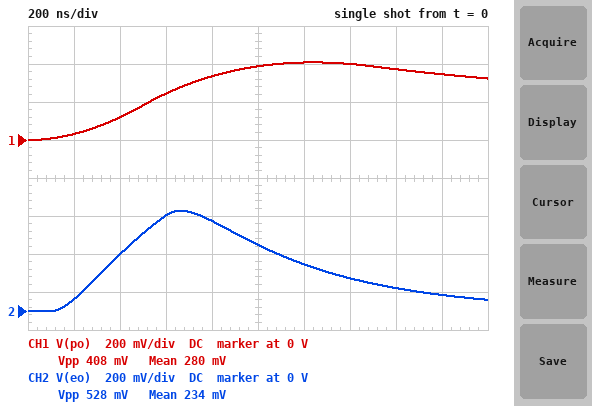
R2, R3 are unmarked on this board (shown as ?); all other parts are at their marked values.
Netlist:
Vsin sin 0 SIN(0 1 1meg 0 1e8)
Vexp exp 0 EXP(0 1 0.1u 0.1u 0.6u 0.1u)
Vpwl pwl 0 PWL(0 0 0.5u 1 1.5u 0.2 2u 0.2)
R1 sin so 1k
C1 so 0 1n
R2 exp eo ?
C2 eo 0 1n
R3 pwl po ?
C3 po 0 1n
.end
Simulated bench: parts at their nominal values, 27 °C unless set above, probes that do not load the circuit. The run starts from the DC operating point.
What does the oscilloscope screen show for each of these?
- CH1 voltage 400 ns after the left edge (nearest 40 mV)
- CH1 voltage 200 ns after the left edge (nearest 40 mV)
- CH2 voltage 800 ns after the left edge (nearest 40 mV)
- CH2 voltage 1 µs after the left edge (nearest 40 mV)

120 mV
40 mV
480 mV
360 mV
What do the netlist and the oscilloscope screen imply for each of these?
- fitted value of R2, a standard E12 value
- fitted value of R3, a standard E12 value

560 Ω
1.2 kΩ
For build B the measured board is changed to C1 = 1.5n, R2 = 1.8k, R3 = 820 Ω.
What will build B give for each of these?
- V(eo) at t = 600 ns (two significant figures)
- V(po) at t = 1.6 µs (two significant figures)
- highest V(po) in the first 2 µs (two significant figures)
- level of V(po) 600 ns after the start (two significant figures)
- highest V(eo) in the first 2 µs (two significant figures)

200 mV
410 mV
500 mV
330 mV
220 mV
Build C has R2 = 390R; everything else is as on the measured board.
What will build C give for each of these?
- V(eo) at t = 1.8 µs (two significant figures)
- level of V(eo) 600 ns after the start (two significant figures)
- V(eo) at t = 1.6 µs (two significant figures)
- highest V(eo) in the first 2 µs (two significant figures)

45 mV
630 mV
75 mV
650 mV
